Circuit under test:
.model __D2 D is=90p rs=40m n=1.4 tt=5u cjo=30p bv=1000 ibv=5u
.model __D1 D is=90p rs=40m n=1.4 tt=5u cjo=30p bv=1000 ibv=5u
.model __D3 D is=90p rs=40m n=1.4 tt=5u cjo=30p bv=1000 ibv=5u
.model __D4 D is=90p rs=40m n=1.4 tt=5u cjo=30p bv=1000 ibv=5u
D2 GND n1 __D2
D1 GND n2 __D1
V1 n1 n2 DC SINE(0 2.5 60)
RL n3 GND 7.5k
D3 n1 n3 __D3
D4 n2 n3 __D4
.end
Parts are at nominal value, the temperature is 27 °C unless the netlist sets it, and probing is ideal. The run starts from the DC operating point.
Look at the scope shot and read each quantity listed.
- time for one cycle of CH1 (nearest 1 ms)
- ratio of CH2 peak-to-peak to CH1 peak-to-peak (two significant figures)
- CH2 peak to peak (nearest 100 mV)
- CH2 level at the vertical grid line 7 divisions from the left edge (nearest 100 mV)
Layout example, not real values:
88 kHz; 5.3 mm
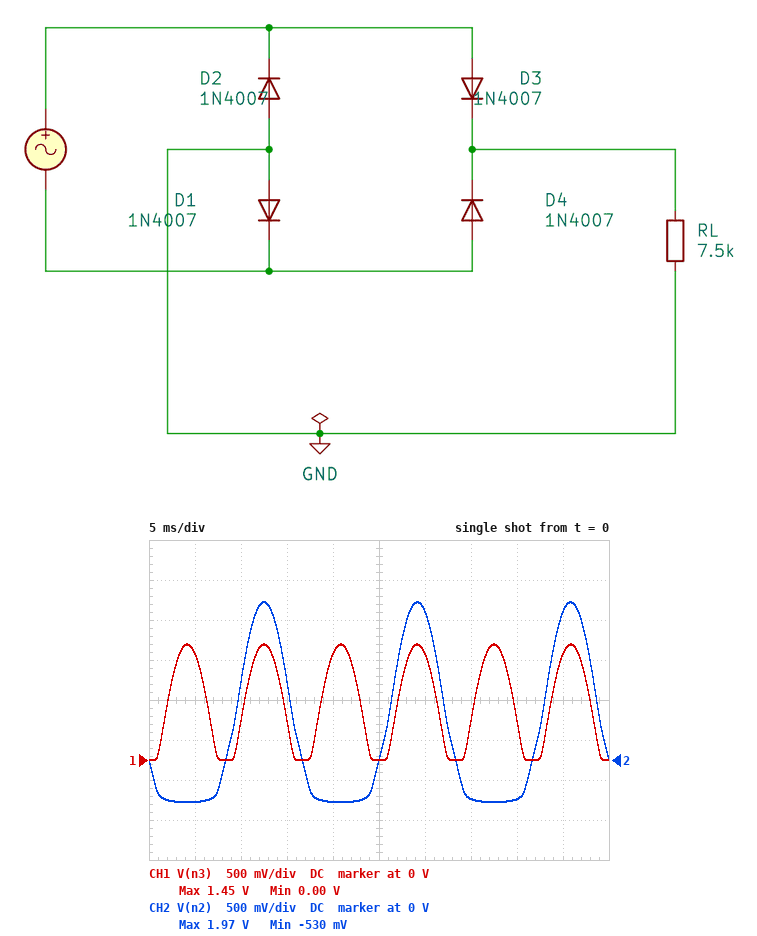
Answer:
8 ms; 1.7; 2.5 V; -500 mV
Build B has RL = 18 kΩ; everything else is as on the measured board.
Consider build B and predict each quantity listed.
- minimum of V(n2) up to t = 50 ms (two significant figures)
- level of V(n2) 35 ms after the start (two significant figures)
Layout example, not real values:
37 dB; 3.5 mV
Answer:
-500 mV; -460 mV
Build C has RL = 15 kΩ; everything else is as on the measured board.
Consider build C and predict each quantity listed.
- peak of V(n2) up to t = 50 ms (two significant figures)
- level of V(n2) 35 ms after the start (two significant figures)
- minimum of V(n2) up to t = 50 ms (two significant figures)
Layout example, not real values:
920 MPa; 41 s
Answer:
2.0 V; -470 mV; -500 mV
